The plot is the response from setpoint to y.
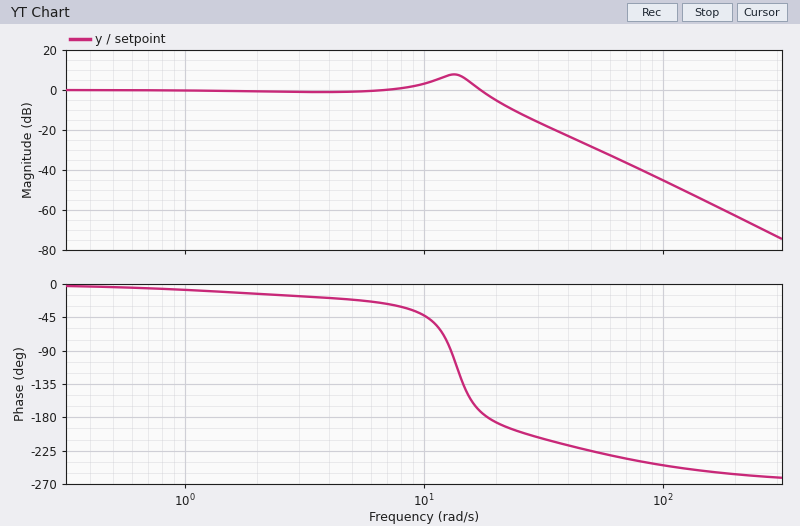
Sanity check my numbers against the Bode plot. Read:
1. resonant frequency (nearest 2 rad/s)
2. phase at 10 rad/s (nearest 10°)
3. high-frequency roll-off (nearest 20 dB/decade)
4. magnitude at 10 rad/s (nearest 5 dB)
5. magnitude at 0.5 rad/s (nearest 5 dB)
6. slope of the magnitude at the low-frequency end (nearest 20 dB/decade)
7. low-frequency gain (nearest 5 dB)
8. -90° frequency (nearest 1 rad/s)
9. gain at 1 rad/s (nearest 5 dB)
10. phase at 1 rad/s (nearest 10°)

14 rad/s
-40°
-60 dB/decade
5 dB
0 dB
0 dB/decade
0 dB
13 rad/s
0 dB
-10°
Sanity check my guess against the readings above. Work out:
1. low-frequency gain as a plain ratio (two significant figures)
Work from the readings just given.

1.0
